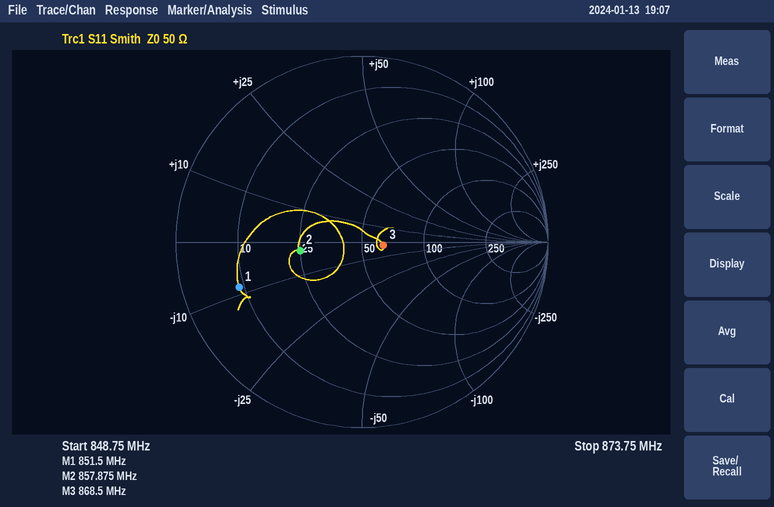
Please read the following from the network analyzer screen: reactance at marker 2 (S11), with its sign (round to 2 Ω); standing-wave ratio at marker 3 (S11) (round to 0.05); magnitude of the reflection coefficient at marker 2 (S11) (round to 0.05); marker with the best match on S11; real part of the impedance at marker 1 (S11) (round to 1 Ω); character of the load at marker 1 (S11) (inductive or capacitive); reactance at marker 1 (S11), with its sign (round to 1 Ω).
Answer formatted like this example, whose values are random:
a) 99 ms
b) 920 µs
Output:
a) -2 Ω
b) 1.25
c) 0.35
d) marker 3
e) 9 Ω
f) capacitive
g) -9 Ω
